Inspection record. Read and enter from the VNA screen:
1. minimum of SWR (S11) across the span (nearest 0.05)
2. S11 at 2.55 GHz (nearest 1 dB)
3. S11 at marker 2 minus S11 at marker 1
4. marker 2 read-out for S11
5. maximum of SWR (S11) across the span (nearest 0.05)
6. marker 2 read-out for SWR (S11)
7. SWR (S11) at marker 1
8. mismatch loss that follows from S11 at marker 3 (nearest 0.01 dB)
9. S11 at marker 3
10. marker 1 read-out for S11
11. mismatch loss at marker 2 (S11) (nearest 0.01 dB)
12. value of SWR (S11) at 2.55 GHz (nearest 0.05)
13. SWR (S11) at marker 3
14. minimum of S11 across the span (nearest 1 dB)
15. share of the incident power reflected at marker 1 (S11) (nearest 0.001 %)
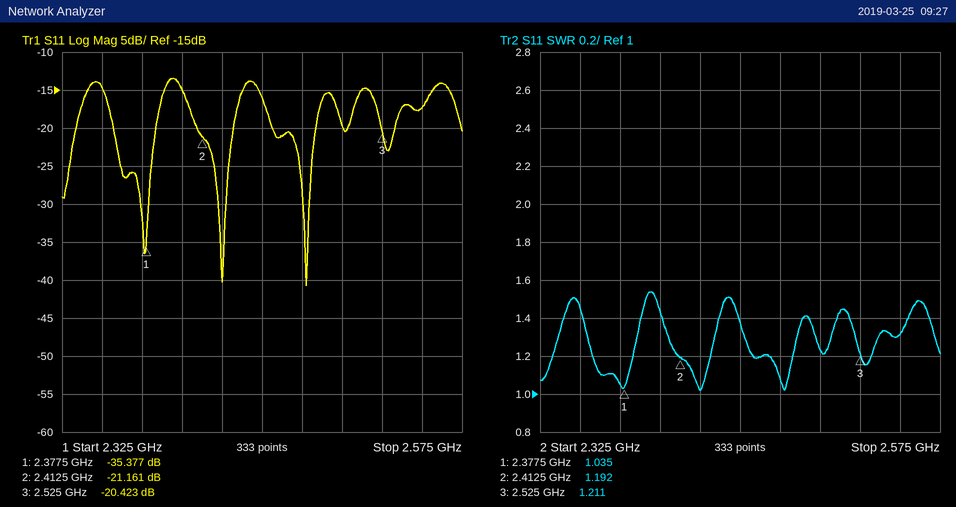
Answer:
1.00
-17 dB
14.216 dB
-21.161 dB
1.55
1.192
1.035
0.04 dB
-20.423 dB
-35.377 dB
0.03 dB
1.30
1.211
-41 dB
0.029 %
